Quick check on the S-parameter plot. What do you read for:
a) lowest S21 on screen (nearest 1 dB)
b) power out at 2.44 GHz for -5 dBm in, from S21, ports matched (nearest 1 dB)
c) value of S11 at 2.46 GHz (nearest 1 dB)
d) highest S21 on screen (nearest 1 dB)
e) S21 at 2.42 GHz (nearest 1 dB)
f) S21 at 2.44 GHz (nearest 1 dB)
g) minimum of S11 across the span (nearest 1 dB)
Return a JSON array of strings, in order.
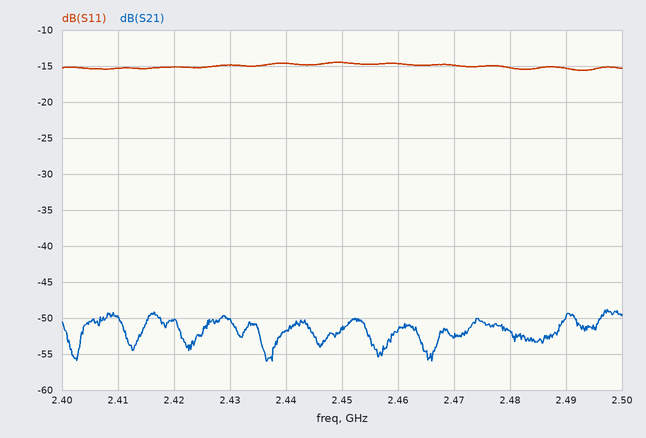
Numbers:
["-56 dB", "-57 dBm", "-15 dB", "-49 dB", "-50 dB", "-52 dB", "-16 dB"]
